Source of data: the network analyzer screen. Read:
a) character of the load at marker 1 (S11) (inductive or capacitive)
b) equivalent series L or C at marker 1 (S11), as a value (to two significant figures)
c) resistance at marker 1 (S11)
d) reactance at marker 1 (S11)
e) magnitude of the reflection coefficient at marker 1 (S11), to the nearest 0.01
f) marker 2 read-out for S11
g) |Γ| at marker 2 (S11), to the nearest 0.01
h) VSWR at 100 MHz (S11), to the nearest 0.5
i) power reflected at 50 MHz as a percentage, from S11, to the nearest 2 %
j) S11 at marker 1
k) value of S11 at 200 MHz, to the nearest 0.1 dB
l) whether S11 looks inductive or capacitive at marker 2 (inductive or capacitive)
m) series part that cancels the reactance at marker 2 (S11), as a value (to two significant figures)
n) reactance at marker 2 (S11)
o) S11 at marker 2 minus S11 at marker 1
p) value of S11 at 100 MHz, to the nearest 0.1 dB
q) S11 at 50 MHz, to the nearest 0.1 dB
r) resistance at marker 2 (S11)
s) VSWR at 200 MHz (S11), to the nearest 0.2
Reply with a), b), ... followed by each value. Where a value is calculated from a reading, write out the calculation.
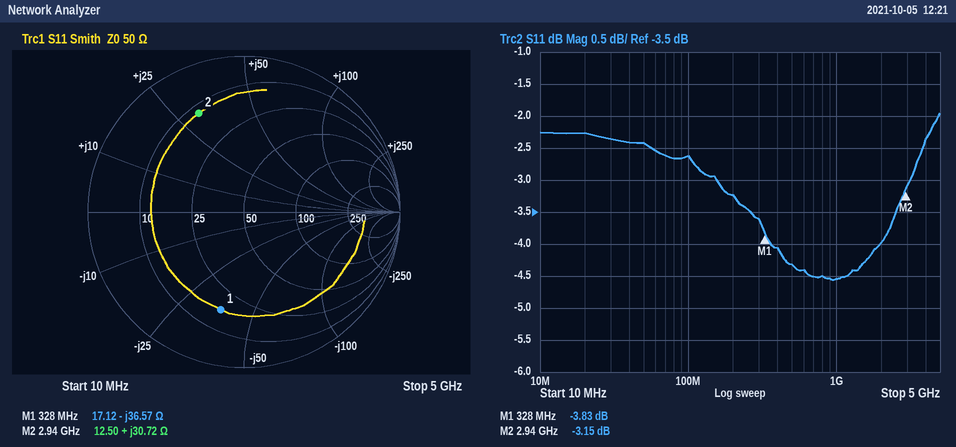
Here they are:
a) capacitive
b) C = 1/(2π × 328 MHz × 36.57 Ω) ≈ 13 pF
c) 17.12 Ω
d) -36.57 Ω
e) 0.64
f) -3.15 dB
g) 0.70
h) |Γ| = 10^(-2.6/20) = 0.7413; VSWR = (1 + 0.7413)/(1 − 0.7413) ≈ 6.73, so 6.5 to the nearest 0.5
i) 10^(-2.4/10) ≈ 58 %
j) -3.83 dB
k) -3.2 dB
l) inductive
m) C = 1/(2π × 2.94 GHz × 30.72 Ω) ≈ 1.8 pF
n) +30.72 Ω
o) -3.15 − (-3.83) = 0.68 dB
p) -2.6 dB
q) -2.4 dB
r) 12.50 Ω
s) |Γ| = 10^(-3.2/20) = 0.6918; VSWR = (1 + 0.6918)/(1 − 0.6918) ≈ 5.49, so 5.4 to the nearest 0.2
